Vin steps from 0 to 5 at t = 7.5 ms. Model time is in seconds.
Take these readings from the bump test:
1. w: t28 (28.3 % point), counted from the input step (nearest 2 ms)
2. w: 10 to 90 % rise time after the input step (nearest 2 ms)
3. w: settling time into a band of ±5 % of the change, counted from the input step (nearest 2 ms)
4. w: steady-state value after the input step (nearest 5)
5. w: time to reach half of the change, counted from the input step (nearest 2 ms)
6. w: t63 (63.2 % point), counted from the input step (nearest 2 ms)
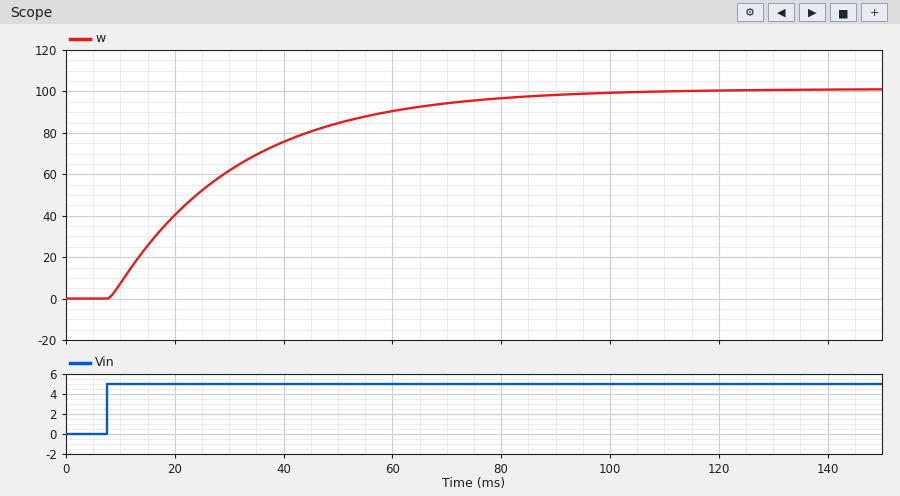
8 ms
50 ms
70 ms
100
16 ms
24 ms
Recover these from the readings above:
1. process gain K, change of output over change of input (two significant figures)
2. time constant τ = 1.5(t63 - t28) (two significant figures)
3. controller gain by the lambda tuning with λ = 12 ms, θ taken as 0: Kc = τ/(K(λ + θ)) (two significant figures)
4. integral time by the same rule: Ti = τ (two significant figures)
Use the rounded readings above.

20
24 ms
0.10
24 ms
